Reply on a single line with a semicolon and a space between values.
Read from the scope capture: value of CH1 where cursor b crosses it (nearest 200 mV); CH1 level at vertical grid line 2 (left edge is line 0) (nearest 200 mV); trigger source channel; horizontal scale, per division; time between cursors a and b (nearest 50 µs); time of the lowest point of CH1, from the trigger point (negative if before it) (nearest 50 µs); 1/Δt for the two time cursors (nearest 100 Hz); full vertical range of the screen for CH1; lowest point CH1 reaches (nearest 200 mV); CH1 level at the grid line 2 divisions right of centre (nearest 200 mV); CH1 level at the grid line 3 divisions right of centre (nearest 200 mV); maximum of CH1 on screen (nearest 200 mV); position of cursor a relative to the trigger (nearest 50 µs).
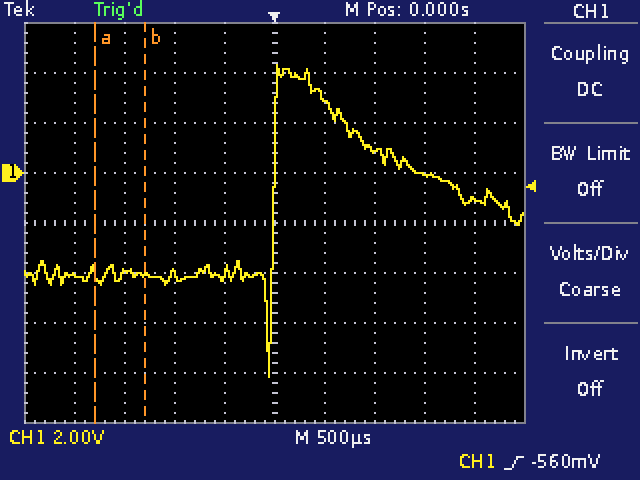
-4.0 V; -4.0 V; CH1; 500 µs; 500 µs; -50 µs; 2.0 kHz; 16 V; -8.2 V; 1.0 V; 0.0 V; 4.4 V; -1.80 ms
